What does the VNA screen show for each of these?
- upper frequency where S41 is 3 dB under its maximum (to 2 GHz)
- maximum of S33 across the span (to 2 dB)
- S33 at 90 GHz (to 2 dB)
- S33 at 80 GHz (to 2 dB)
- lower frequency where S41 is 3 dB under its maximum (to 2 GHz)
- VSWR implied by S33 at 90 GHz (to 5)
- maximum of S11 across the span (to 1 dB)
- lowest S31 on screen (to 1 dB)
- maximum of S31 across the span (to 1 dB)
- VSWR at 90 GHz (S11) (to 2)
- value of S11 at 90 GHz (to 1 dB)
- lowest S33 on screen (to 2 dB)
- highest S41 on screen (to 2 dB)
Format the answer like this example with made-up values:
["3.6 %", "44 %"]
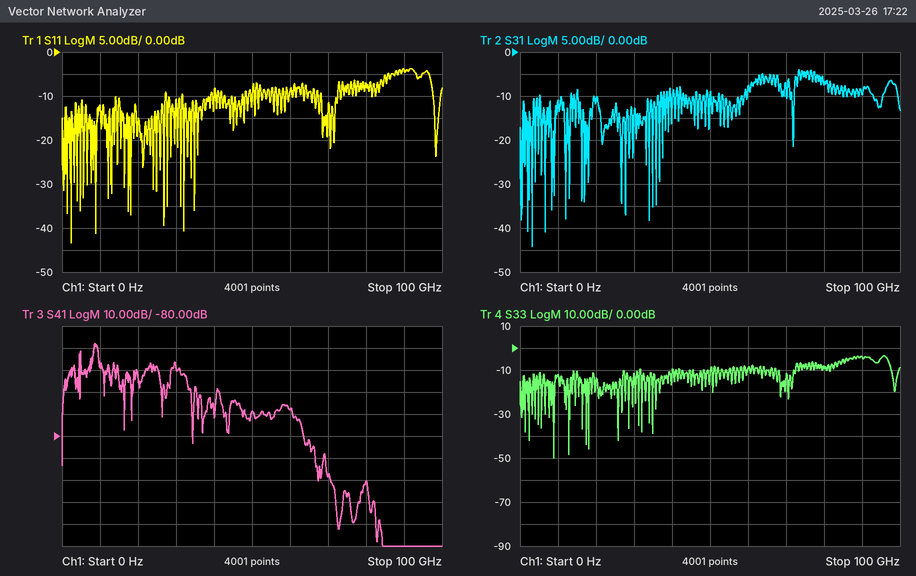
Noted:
["10 GHz", "-4 dB", "-4 dB", "-8 dB", "8 GHz", "5", "-4 dB", "-44 dB", "-4 dB", "4", "-4 dB", "-50 dB", "-38 dB"]
